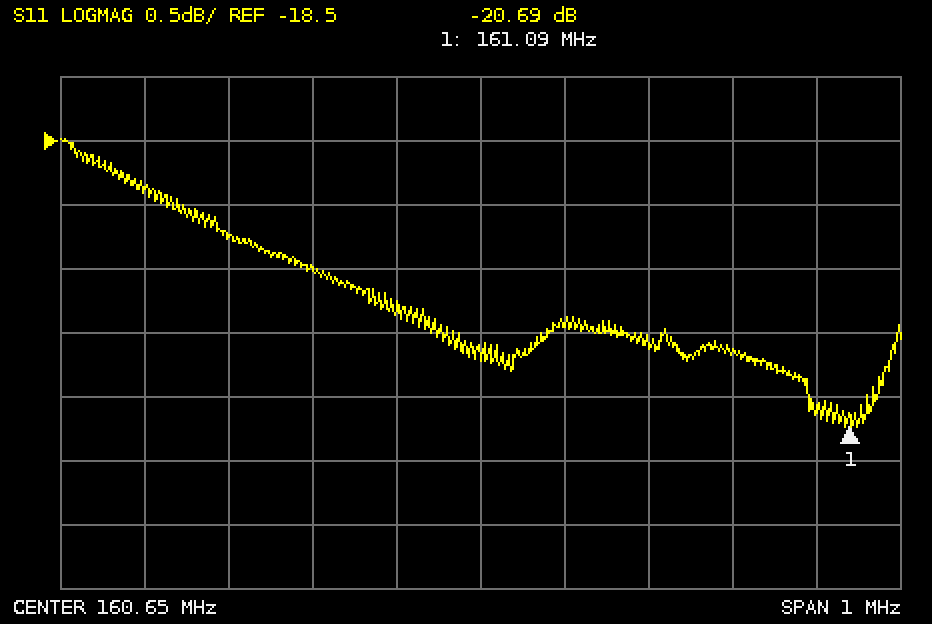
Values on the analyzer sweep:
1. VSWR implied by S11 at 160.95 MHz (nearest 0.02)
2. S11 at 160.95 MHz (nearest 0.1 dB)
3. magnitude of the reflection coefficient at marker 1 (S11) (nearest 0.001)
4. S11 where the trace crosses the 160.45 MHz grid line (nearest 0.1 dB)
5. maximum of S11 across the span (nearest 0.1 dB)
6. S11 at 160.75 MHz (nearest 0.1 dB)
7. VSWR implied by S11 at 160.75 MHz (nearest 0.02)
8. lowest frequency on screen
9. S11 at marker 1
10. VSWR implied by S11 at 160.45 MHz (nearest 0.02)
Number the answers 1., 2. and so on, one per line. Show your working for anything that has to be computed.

1. |Γ| = 10^(-20.1/20) = 0.0989; VSWR = (1 + 0.0989)/(1 − 0.0989) ≈ 1.22
2. -20.1 dB
3. 10^(-20.69/20) ≈ 0.092
4. -19.5 dB
5. -18.5 dB
6. -19.9 dB
7. |Γ| = 10^(-19.9/20) = 0.1012; VSWR = (1 + 0.1012)/(1 − 0.1012) ≈ 1.23, so 1.22 to the nearest 0.02
8. 160.15 MHz
9. -20.69 dB
10. |Γ| = 10^(-19.5/20) = 0.1059; VSWR = (1 + 0.1059)/(1 − 0.1059) ≈ 1.24
